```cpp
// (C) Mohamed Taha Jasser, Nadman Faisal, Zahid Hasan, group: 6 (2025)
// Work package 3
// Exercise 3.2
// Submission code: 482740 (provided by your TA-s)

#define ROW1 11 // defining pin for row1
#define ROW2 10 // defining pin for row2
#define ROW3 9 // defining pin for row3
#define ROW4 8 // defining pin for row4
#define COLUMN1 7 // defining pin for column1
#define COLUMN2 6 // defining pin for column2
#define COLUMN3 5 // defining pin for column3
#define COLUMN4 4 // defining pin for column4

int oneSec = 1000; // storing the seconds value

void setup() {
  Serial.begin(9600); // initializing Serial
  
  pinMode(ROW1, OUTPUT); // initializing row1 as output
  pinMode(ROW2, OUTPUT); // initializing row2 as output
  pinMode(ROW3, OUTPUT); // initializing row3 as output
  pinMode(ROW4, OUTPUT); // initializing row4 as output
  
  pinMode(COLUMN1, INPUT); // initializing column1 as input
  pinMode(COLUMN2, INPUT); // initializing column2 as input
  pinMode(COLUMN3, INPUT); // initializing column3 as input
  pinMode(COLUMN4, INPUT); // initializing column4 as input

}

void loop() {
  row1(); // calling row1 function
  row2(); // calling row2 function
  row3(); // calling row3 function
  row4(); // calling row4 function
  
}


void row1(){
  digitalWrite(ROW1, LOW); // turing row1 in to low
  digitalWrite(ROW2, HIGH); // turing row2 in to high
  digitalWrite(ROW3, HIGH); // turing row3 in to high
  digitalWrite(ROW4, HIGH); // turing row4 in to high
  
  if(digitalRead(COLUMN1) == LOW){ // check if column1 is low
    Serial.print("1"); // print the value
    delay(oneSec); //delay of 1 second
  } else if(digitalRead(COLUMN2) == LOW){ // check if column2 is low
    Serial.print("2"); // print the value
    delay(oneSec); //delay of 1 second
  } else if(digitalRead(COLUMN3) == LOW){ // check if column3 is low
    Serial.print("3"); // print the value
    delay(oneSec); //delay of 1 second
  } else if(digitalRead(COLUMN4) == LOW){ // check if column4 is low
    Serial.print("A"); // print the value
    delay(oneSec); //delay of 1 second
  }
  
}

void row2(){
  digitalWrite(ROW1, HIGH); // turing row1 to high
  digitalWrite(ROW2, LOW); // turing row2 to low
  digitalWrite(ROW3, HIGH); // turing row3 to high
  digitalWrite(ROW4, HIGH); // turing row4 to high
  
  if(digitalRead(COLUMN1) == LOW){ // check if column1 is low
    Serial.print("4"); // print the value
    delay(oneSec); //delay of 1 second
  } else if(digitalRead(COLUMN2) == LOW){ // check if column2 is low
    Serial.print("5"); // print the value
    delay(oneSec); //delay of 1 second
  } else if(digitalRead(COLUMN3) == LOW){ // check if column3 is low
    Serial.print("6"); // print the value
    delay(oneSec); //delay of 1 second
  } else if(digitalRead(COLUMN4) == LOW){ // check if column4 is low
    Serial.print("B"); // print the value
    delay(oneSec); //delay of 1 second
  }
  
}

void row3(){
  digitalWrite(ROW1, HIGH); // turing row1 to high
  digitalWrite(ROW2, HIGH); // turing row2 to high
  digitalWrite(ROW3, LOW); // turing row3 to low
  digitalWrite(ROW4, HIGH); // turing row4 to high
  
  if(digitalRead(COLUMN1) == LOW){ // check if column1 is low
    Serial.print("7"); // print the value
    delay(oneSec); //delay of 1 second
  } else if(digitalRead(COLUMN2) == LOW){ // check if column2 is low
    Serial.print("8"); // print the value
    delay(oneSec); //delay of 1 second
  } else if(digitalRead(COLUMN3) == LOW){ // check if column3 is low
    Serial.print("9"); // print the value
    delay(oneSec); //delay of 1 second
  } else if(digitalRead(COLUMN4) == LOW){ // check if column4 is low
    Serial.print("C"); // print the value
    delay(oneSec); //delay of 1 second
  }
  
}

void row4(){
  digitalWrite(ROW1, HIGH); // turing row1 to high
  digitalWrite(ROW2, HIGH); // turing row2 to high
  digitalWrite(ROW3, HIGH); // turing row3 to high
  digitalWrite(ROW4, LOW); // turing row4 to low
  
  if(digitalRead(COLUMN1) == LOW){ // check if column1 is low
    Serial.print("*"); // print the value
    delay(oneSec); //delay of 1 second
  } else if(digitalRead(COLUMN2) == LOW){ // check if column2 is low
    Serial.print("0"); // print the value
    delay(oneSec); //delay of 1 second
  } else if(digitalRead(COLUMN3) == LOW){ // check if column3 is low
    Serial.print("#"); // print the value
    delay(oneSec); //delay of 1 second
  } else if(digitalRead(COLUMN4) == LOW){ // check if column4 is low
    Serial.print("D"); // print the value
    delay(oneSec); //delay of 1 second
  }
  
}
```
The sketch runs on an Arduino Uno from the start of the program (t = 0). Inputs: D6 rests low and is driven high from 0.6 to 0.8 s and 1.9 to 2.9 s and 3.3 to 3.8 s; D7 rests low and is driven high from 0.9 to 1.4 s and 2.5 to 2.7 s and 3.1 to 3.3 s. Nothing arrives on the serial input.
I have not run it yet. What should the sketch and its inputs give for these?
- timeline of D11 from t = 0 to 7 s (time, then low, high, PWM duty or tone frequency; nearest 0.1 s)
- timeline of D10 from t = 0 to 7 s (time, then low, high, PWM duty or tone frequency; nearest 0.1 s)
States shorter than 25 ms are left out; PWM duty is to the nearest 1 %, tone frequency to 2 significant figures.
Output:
0 s low; 1 s high; 4 s low; 5 s high
0 s high; 1 s low; 2 s high; 5 s low; 6 s high
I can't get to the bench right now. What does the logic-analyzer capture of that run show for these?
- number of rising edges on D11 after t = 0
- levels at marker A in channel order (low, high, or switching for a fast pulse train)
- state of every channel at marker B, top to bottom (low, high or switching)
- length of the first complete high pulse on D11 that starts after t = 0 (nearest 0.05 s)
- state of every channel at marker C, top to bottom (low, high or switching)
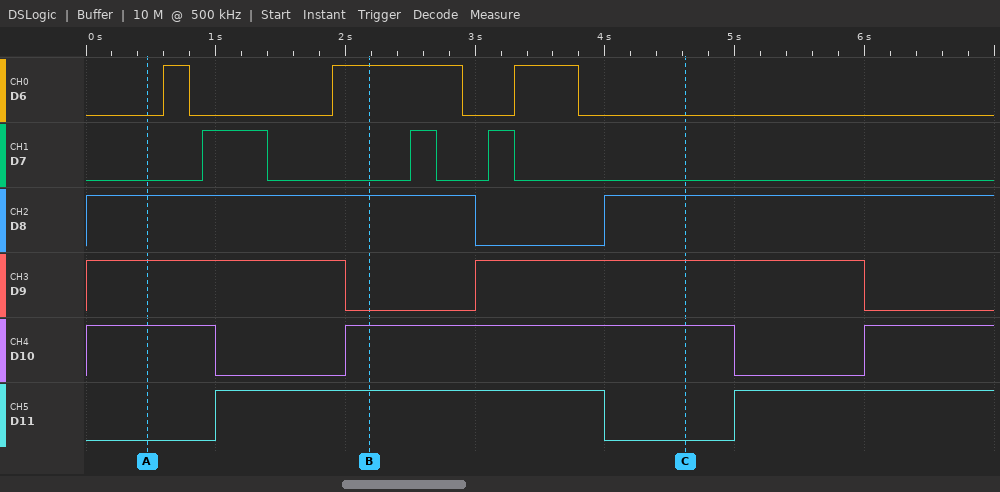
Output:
2
D6 low, D7 low, D8 high, D9 high, D10 high, D11 low
D6 high, D7 low, D8 high, D9 low, D10 high, D11 high
3.00 s
D6 low, D7 low, D8 high, D9 high, D10 high, D11 low
